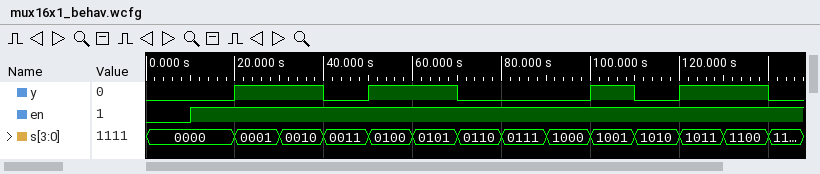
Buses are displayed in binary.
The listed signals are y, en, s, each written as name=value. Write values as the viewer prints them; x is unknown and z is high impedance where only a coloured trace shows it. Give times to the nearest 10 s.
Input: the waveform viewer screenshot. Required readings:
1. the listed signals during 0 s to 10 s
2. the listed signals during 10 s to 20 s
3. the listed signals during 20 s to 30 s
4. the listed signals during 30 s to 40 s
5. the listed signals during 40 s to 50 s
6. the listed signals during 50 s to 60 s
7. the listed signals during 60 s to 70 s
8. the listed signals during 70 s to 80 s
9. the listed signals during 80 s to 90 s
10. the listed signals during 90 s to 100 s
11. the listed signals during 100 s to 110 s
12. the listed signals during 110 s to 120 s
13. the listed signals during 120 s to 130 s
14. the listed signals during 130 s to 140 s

y=0, en=0, s=0000
y=0, en=1, s=0000
y=1, en=1, s=0001
y=1, en=1, s=0010
y=0, en=1, s=0011
y=1, en=1, s=0100
y=1, en=1, s=0101
y=0, en=1, s=0110
y=0, en=1, s=0111
y=0, en=1, s=1000
y=1, en=1, s=1001
y=0, en=1, s=1010
y=1, en=1, s=1011
y=1, en=1, s=1100
